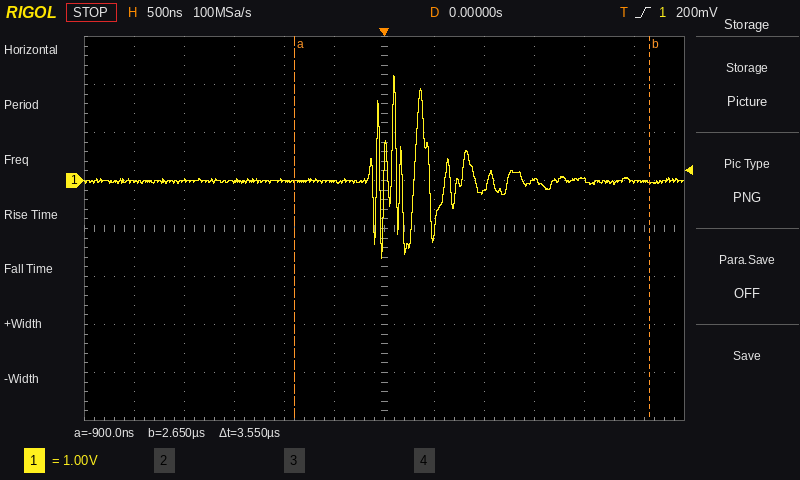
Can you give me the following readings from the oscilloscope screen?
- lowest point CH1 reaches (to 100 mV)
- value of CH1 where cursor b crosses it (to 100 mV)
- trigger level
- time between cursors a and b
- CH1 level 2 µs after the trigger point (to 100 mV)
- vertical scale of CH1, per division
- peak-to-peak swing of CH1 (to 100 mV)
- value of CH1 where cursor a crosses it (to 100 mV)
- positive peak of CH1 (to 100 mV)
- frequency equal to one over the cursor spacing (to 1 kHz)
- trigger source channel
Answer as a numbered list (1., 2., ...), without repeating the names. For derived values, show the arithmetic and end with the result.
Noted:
1. -1.6 V
2. 0.0 V
3. 200 mV
4. 3.55 µs
5. 0.0 V
6. 1 V
7. 2.2 V − (-1.6 V) = 3.8 V
8. 0.0 V
9. 2.2 V
10. 1 / 3.55 µs ≈ 282 kHz
11. CH1
